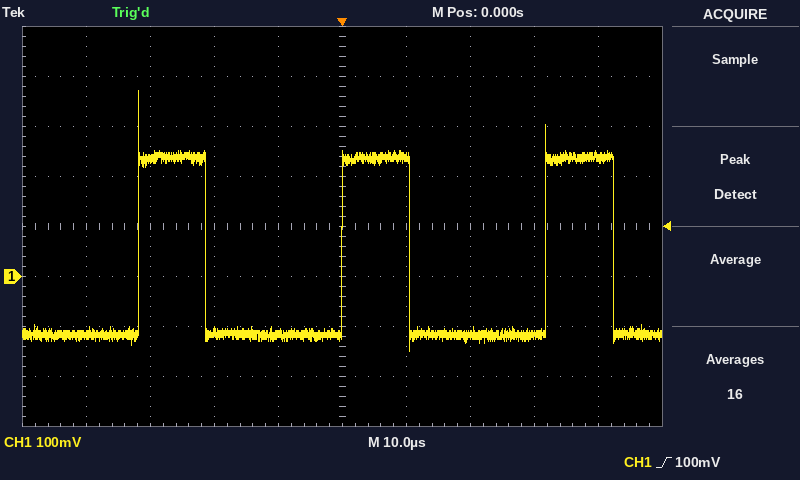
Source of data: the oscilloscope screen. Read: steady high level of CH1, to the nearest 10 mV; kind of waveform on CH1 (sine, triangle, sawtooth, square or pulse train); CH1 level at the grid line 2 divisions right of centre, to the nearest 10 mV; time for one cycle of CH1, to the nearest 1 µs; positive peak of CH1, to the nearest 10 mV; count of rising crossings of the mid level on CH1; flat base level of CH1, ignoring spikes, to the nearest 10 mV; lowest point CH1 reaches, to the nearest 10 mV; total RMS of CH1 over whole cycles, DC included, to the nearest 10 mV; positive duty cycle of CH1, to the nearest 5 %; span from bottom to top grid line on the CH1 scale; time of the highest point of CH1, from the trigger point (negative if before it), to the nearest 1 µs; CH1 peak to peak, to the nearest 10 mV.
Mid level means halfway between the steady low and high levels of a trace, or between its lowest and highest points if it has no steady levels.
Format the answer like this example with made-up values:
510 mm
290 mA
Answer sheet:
240 mV
pulse train
-120 mV
32 µs
370 mV
3
-120 mV
-150 mV
170 mV
35 %
800 mV
-32 µs
520 mV
